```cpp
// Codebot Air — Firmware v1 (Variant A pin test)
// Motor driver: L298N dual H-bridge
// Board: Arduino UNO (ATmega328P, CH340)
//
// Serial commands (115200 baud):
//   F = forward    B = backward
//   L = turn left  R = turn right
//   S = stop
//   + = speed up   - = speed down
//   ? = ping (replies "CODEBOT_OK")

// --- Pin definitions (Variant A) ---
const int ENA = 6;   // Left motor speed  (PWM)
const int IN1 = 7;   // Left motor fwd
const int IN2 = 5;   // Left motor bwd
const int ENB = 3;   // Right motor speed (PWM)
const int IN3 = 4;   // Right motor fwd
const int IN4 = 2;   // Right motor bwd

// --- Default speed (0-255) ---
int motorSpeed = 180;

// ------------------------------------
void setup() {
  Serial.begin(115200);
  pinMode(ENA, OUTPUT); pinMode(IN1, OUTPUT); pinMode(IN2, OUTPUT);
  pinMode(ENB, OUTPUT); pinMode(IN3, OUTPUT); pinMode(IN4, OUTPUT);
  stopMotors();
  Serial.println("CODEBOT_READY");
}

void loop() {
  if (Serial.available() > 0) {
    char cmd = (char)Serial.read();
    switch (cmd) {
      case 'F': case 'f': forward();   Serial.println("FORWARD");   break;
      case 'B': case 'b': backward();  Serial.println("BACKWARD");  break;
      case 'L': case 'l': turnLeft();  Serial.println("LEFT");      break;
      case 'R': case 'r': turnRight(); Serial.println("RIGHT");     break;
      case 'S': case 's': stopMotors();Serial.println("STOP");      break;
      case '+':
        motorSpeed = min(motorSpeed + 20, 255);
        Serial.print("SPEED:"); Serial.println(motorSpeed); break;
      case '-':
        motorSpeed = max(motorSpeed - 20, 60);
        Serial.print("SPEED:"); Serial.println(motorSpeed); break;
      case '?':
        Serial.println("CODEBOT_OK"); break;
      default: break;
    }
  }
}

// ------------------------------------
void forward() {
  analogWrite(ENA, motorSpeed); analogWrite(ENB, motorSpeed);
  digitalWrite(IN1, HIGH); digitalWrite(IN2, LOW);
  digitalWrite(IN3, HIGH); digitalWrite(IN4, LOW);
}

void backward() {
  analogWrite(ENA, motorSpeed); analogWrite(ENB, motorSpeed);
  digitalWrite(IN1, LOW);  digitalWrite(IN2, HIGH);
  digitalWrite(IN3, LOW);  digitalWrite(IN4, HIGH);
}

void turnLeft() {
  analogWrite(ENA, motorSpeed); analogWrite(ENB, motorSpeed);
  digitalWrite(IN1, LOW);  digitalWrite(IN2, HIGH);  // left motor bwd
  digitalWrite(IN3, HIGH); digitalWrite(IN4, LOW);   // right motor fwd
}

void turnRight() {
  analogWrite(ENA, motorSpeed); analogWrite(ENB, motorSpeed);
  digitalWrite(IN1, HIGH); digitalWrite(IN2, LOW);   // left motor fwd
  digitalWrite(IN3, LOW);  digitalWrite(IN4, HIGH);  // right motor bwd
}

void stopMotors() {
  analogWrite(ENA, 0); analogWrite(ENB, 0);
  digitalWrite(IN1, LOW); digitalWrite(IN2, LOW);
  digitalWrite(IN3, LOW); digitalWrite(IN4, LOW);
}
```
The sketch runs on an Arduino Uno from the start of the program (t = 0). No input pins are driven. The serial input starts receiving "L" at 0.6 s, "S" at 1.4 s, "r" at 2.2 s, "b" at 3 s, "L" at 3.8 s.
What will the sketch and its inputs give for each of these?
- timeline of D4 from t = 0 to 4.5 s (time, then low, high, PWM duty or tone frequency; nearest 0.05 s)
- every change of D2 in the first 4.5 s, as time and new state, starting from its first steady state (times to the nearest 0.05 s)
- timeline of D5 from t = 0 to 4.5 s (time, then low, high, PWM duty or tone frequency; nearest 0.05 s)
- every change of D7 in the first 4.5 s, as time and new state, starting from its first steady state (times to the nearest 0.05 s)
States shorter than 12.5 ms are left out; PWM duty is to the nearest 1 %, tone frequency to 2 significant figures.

0 s low; 0.6 s high; 1.4 s low; 3.8 s high
0 s low; 2.2 s high; 3.8 s low
0 s low; 0.6 s high; 1.4 s low; 3 s high
0 s low; 2.2 s high; 3 s low
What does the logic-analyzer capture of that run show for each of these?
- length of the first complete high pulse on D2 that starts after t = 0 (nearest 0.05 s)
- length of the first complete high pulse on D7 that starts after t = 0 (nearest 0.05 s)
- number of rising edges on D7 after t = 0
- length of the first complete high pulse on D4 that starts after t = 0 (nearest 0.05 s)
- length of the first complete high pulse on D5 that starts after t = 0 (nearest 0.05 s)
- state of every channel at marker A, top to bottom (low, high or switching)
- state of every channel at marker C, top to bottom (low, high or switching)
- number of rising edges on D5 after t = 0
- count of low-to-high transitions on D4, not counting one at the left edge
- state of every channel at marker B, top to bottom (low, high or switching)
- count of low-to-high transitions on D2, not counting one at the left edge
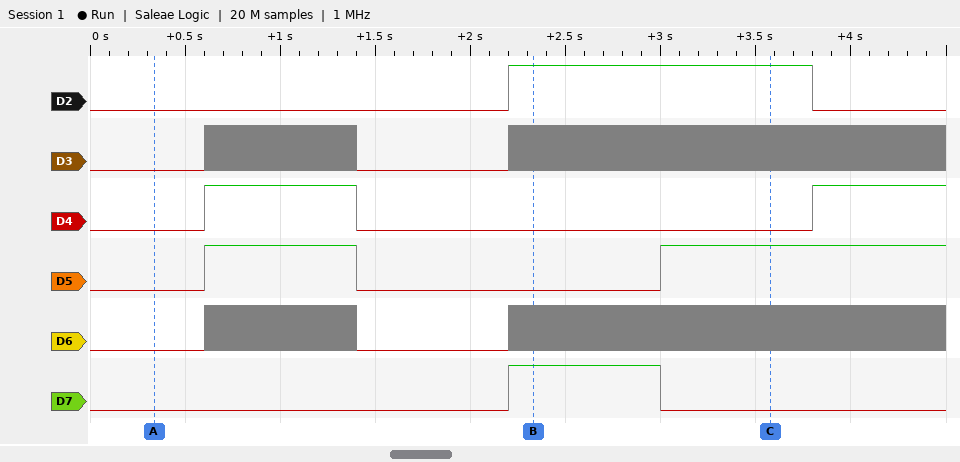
1.60 s
0.80 s
1
0.80 s
0.80 s
D2 low, D3 low, D4 low, D5 low, D6 low, D7 low
D2 high, D3 switching, D4 low, D5 high, D6 switching, D7 low
2
2
D2 high, D3 switching, D4 low, D5 low, D6 switching, D7 high
1
